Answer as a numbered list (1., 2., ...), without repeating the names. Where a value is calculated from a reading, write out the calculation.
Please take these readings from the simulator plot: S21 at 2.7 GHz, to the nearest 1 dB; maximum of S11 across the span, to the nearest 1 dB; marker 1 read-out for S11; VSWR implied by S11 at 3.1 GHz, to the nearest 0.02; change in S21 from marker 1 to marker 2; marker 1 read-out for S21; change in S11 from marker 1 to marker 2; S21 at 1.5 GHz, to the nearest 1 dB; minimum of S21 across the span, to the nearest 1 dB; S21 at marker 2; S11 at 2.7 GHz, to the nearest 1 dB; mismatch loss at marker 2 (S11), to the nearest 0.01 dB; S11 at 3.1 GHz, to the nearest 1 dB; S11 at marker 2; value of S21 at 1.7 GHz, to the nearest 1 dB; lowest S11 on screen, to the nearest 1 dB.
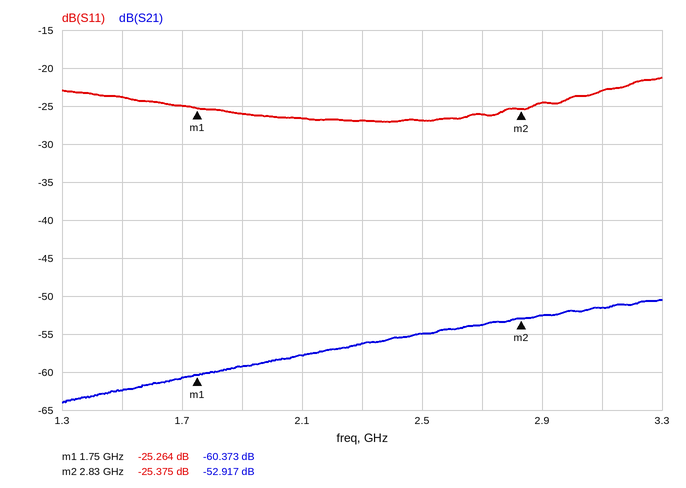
1. -54 dB
2. -21 dB
3. -25.264 dB
4. |Γ| = 10^(-23/20) = 0.0708; VSWR = (1 + 0.0708)/(1 − 0.0708) ≈ 1.15, so 1.16 to the nearest 0.02
5. -52.917 − (-60.373) = 7.456 dB
6. -60.373 dB
7. -25.375 − (-25.264) = -0.111 dB
8. -62 dB
9. -64 dB
10. -52.917 dB
11. -26 dB
12. −10 log10(1 − 10^(-25.375/10)) ≈ 0.01 dB
13. -23 dB
14. -25.375 dB
15. -61 dB
16. -27 dB
